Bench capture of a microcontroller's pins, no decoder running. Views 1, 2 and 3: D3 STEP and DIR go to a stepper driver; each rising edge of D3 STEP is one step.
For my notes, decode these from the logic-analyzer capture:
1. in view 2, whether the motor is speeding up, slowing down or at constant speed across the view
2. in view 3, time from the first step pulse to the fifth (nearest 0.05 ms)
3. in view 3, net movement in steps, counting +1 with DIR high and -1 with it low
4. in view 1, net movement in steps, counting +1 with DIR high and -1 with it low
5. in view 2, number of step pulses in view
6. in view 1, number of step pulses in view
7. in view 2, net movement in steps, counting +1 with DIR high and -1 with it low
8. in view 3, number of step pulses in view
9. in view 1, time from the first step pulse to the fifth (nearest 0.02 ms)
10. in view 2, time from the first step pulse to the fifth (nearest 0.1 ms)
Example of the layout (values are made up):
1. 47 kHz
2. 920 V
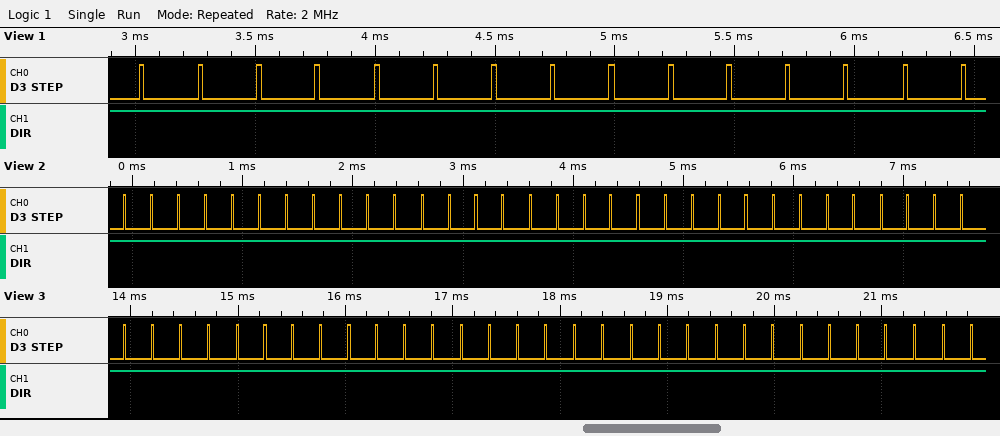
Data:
1. constant speed
2. 1.05 ms
3. +31
4. +15
5. 32
6. 15
7. +32
8. 31
9. 0.98 ms
10. 1.0 ms
